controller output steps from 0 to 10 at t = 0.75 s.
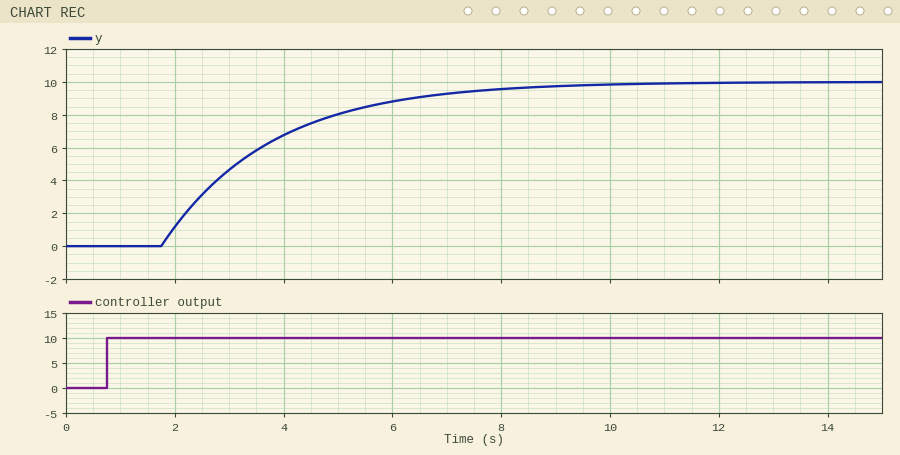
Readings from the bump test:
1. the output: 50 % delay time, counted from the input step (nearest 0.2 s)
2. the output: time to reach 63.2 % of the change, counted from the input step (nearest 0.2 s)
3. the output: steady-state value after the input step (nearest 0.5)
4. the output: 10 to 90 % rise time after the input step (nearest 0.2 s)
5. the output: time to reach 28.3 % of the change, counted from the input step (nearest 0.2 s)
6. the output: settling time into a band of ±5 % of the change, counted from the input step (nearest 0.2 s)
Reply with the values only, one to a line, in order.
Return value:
2.4 s
3.0 s
10.0
4.4 s
1.6 s
7.0 s
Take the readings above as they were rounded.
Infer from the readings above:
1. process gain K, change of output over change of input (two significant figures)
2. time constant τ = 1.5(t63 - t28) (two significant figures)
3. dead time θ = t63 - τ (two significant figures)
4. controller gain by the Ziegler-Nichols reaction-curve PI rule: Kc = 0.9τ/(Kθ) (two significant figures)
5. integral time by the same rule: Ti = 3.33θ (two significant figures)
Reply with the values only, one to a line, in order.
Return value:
1.0
2.1 s
0.90 s
2.1
3.0 s
